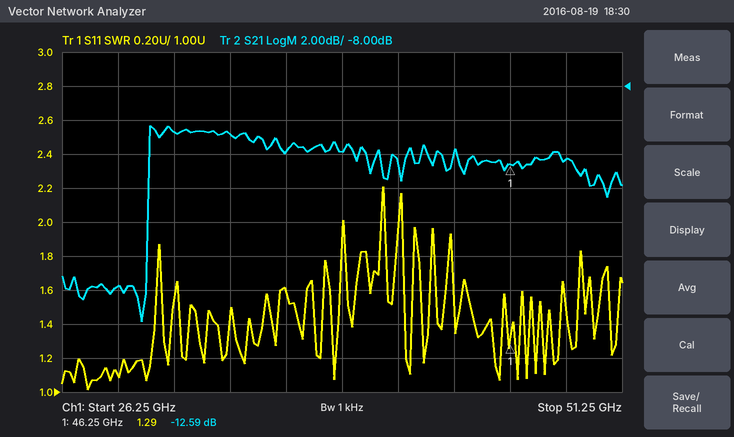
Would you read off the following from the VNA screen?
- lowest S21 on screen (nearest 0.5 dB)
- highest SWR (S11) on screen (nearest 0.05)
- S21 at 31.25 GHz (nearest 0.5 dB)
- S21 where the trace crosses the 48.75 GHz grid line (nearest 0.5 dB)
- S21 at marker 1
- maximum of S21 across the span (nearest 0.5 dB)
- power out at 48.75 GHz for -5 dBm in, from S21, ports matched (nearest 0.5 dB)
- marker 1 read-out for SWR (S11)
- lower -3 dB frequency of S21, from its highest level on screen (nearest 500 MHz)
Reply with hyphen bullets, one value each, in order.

- -22.0 dB
- 2.20
- -10.5 dB
- -12.5 dB
- -12.59 dB
- -10.5 dB
- -17.5 dBm
- 1.29
- 30.0 GHz
